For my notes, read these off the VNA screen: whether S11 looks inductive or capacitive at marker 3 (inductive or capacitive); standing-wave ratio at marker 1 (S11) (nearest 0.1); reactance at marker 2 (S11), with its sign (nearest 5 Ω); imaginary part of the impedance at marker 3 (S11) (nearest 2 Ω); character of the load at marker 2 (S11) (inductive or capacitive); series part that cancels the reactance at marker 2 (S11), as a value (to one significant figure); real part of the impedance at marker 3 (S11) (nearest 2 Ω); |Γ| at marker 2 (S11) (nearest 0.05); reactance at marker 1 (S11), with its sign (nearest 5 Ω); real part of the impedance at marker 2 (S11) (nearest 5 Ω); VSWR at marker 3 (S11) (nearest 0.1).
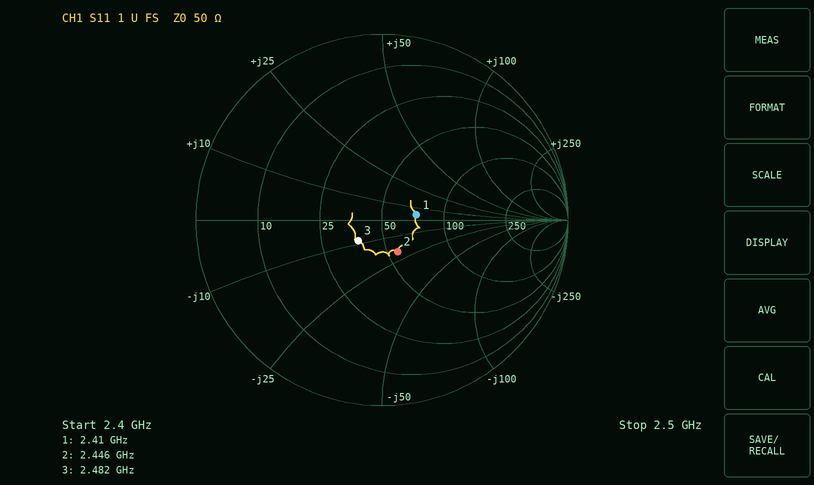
capacitive
1.5
-20 Ω
-8 Ω
capacitive
1 nH
38 Ω
0.20
+5 Ω
55 Ω
1.4
